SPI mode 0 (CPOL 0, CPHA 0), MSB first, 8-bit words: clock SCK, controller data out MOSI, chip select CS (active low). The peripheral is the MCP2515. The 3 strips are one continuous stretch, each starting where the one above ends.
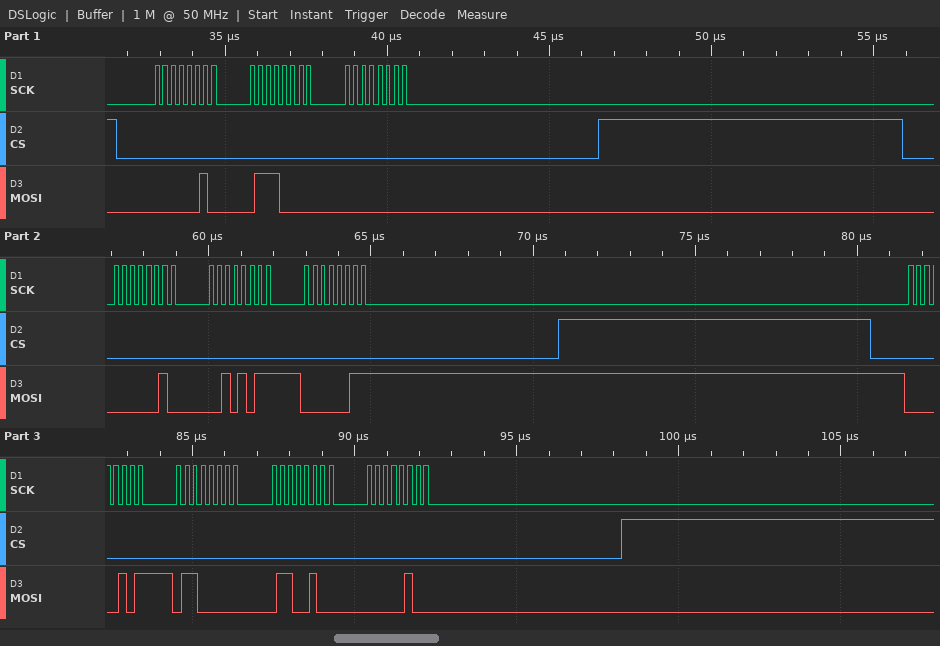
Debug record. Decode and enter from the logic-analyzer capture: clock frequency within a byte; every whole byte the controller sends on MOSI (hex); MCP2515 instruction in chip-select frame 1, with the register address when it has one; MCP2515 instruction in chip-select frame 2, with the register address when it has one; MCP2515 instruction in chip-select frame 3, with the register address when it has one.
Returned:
4 MHz
02 70 00 02 2B 03 05 60 64 04
WRITE 0x70
WRITE 0x2B
BIT MODIFY 0x60
